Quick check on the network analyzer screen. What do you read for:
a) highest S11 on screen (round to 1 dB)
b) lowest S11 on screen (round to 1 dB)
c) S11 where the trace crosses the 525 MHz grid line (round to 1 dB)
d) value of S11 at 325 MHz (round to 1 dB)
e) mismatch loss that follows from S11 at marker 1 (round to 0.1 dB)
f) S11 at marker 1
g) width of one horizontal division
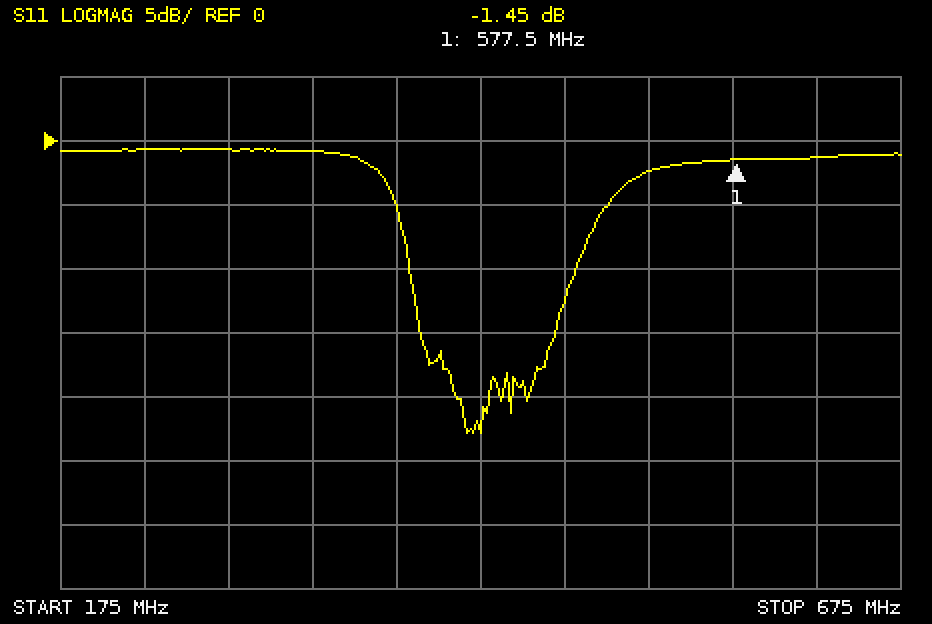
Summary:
-1 dB
-23 dB
-2 dB
-1 dB
5.5 dB
-1.45 dB
50 MHz
